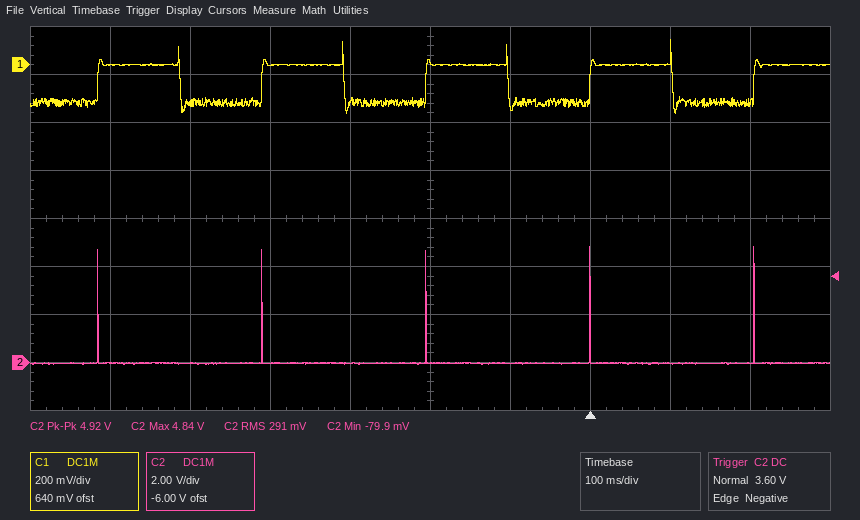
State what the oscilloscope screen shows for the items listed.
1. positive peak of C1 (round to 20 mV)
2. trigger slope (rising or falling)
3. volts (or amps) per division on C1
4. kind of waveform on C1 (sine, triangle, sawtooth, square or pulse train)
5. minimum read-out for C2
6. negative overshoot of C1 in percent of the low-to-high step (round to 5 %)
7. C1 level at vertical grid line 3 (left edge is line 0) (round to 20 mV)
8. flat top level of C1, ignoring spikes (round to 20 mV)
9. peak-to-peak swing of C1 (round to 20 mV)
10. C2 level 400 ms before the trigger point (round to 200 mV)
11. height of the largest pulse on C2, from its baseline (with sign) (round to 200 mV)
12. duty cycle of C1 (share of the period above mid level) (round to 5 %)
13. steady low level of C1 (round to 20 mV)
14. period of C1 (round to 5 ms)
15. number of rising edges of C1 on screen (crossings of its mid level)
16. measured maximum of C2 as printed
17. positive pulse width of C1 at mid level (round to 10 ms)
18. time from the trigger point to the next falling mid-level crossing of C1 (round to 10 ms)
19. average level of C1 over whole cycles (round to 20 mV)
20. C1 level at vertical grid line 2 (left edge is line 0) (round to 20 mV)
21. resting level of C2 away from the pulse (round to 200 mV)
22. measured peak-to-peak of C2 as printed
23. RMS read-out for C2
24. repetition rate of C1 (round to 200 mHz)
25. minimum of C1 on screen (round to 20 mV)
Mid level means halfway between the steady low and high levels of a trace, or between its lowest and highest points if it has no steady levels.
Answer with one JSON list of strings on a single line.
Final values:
["100 mV", "falling", "200 mV", "square", "-79.9 mV", "30 %", "0 mV", "0 mV", "300 mV", "0.0 V", "+4.8 V", "50 %", "-160 mV", "205 ms", "5", "4.84 V", "100 ms", "100 ms", "-80 mV", "-160 mV", "0.0 V", "4.92 V", "291 mV", "4.8 Hz", "-200 mV"]
